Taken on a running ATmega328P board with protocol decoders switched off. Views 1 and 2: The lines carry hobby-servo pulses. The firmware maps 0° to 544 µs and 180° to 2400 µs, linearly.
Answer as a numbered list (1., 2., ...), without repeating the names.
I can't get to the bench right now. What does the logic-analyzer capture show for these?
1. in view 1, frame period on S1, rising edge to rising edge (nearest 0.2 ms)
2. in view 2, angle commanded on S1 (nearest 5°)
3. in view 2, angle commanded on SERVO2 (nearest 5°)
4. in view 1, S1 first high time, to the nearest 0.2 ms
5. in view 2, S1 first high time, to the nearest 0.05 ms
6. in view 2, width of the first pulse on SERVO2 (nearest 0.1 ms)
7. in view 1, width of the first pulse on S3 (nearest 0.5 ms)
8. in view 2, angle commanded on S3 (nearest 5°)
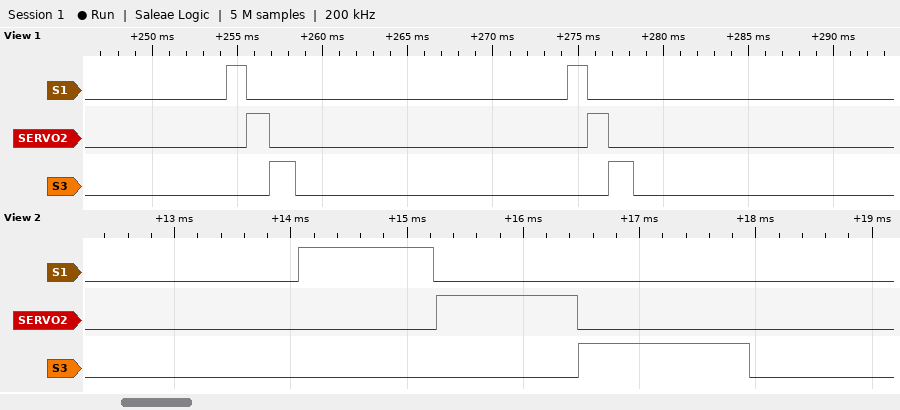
1. 20.0 ms
2. 60°
3. 65°
4. 1.2 ms
5. 1.15 ms
6. 1.2 ms
7. 1.5 ms
8. 90°
